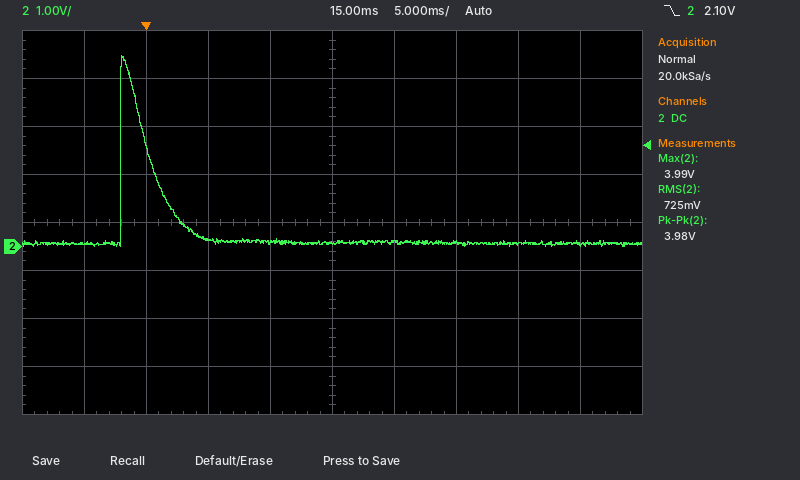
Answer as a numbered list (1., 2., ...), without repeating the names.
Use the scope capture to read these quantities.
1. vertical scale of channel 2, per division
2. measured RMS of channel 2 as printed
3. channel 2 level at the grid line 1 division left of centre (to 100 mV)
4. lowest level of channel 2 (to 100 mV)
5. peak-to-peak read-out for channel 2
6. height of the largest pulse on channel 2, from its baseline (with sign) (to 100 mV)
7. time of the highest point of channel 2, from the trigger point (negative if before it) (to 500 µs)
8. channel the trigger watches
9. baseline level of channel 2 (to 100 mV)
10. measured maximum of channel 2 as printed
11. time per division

1. 1 V
2. 725 mV
3. 100 mV
4. 0.0 V
5. 3.98 V
6. +3.9 V
7. -2.0 ms
8. channel 2
9. 100 mV
10. 3.99 V
11. 5 ms
